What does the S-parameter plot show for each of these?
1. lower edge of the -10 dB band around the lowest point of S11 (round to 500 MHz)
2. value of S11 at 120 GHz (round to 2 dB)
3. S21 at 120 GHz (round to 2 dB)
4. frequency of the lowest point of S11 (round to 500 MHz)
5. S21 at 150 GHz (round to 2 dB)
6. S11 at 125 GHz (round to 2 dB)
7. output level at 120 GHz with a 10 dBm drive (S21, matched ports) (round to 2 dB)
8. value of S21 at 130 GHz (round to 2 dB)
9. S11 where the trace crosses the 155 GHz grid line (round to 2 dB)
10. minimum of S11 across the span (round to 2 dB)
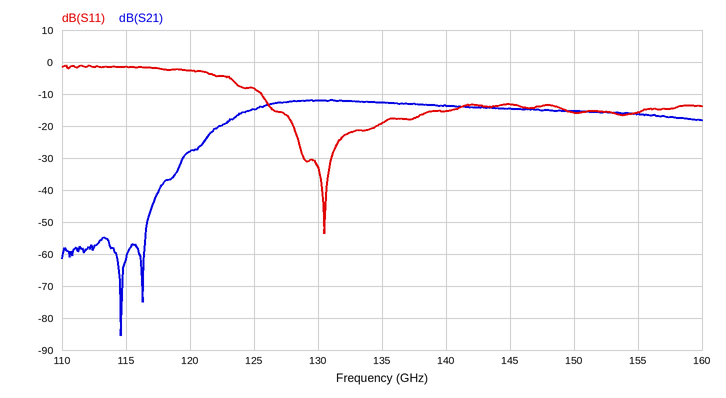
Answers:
125.5 GHz
-2 dB
-28 dB
130.5 GHz
-16 dB
-8 dB
-18 dBm
-12 dB
-16 dB
-54 dB
